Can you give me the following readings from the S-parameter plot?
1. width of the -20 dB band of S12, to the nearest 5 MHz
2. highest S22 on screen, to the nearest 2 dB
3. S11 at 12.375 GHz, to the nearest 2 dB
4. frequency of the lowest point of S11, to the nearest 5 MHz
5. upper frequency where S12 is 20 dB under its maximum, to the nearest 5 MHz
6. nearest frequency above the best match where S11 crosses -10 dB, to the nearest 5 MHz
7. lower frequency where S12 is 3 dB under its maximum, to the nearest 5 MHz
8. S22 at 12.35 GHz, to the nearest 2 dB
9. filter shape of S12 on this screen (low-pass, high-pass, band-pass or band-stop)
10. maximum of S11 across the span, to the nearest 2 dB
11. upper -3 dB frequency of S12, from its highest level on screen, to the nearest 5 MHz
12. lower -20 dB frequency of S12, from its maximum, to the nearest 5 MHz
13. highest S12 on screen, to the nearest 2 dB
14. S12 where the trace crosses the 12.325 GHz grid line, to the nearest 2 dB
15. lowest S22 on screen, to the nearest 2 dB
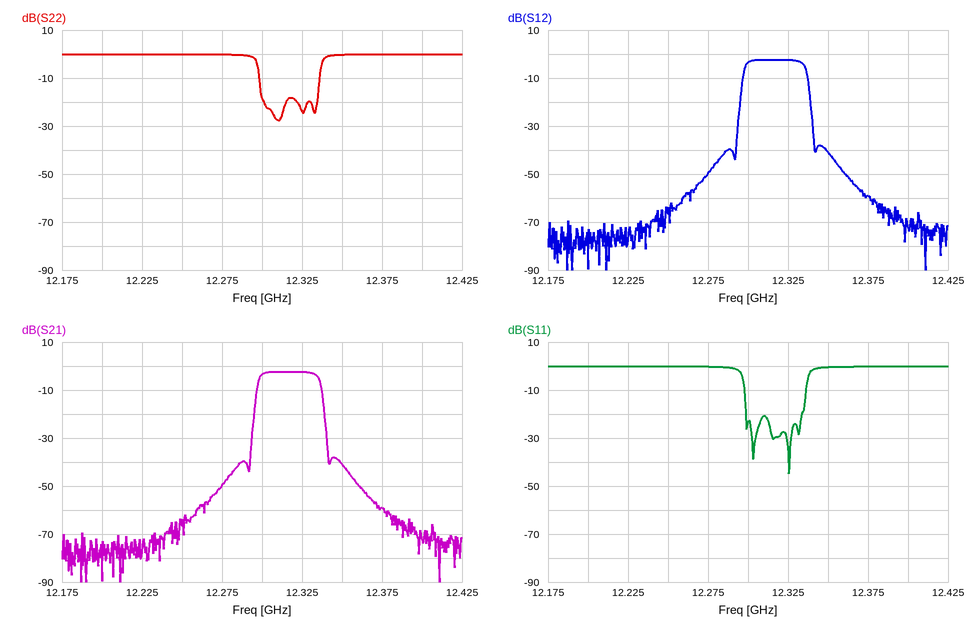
45 MHz
0 dB
0 dB
12.325 GHz
12.340 GHz
12.335 GHz
12.300 GHz
0 dB
band-pass
0 dB
12.335 GHz
12.295 GHz
-2 dB
-2 dB
-28 dB
